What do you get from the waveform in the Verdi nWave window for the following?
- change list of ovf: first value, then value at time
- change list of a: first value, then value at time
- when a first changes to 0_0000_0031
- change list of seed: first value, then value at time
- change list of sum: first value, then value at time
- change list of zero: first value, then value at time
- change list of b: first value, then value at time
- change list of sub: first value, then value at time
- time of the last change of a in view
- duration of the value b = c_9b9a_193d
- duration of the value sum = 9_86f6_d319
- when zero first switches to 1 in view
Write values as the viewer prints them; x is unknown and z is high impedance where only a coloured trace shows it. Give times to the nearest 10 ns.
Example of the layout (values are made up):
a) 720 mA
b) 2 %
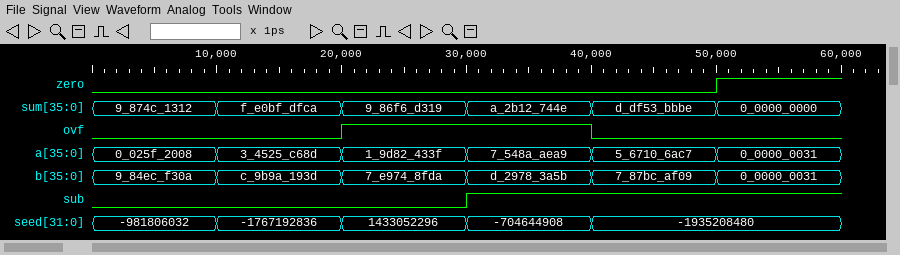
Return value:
a) 0, 1 at 20 ns, 0 at 40 ns
b) 0_025f_2008, 3_4525_c68d at 10 ns, 1_9d82_433f at 20 ns, 7_548a_aea9 at 30 ns, 5_6710_6ac7 at 40 ns, 0_0000_0031 at 50 ns
c) 50 ns
d) -981806032, -1767192836 at 10 ns, 1433052296 at 20 ns, -704644908 at 30 ns, -1935208480 at 40 ns
e) 9_874c_1312, f_e0bf_dfca at 10 ns, 9_86f6_d319 at 20 ns, a_2b12_744e at 30 ns, d_df53_bbbe at 40 ns, 0_0000_0000 at 50 ns
f) 0, 1 at 50 ns
g) 9_84ec_f30a, c_9b9a_193d at 10 ns, 7_e974_8fda at 20 ns, d_2978_3a5b at 30 ns, 7_87bc_af09 at 40 ns, 0_0000_0031 at 50 ns
h) 0, 1 at 30 ns
i) 50 ns
j) 10 ns
k) 10 ns
l) 50 ns
